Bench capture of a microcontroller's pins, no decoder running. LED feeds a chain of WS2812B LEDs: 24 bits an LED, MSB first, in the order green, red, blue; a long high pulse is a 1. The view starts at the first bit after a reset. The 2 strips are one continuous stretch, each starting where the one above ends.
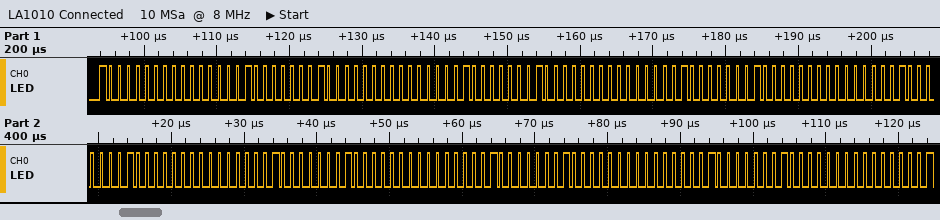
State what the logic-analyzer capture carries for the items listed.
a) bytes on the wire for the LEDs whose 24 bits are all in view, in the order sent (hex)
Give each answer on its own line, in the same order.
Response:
80 00 80 80 00 80 80 00 80 80 00 80 80 00 80 80 00 80 80 00 80
